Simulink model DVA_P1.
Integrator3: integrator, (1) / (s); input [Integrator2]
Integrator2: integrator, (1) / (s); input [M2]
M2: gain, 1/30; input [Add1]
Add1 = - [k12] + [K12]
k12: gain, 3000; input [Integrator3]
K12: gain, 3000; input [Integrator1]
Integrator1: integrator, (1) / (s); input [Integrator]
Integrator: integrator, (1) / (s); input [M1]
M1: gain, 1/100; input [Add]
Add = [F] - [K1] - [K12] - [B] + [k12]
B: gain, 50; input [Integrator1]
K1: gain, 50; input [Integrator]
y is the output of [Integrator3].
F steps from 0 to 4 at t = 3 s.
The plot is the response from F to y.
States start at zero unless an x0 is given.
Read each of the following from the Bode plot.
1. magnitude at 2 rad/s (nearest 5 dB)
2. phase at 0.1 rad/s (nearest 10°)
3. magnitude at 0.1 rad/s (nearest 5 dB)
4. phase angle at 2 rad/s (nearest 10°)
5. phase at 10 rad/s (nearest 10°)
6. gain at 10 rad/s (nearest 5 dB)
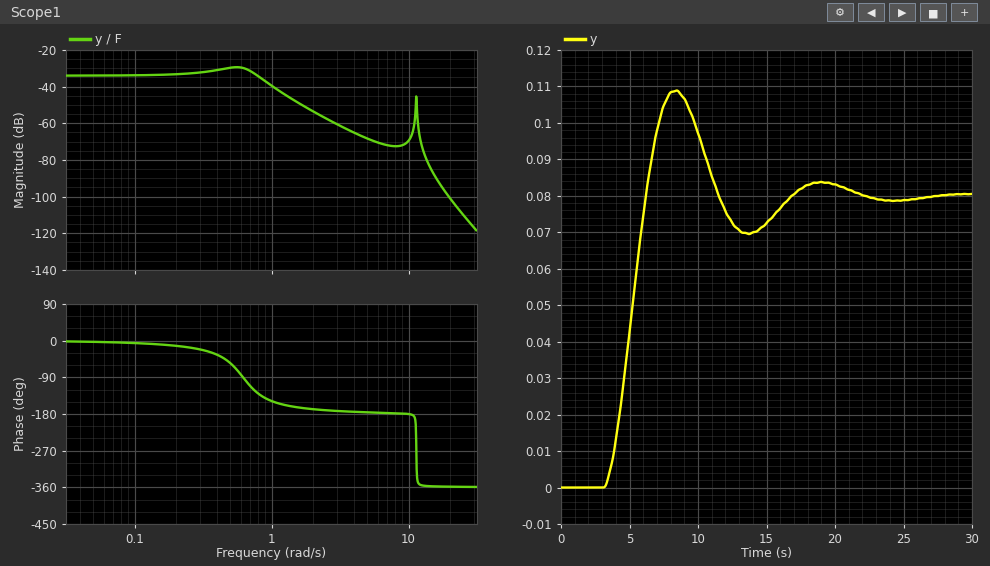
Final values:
-55 dB
-10°
-35 dB
-170°
-180°
-70 dB
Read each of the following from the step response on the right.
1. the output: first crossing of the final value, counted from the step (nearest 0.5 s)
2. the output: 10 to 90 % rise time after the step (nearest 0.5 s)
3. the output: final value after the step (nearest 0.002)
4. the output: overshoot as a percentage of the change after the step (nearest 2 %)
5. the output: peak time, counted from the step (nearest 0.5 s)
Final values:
3.0 s
2.0 s
0.080
36 %
5.5 s
